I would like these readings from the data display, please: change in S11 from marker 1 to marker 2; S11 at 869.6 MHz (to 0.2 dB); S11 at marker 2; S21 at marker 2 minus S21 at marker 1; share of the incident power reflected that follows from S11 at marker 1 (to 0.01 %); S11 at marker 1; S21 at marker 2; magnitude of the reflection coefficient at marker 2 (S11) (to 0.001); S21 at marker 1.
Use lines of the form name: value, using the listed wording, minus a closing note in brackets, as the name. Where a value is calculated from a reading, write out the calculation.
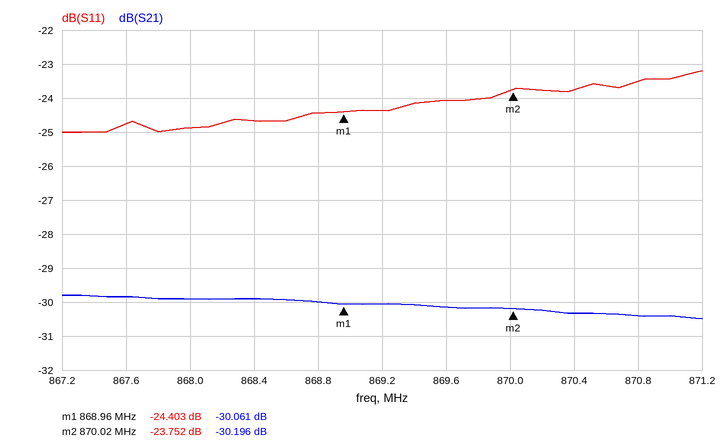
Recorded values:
change in S11 from marker 1 to marker 2: -23.752 − (-24.403) = 0.651 dB
S11 at 869.6 MHz: -24.0 dB
S11 at marker 2: -23.752 dB
S21 at marker 2 minus S21 at marker 1: -30.196 − (-30.061) = -0.135 dB
share of the incident power reflected that follows from S11 at marker 1: 10^(-24.403/10) ≈ 0.36 %
S11 at marker 1: -24.403 dB
S21 at marker 2: -30.196 dB
magnitude of the reflection coefficient at marker 2 (S11): 10^(-23.752/20) ≈ 0.065
S21 at marker 1: -30.061 dB
